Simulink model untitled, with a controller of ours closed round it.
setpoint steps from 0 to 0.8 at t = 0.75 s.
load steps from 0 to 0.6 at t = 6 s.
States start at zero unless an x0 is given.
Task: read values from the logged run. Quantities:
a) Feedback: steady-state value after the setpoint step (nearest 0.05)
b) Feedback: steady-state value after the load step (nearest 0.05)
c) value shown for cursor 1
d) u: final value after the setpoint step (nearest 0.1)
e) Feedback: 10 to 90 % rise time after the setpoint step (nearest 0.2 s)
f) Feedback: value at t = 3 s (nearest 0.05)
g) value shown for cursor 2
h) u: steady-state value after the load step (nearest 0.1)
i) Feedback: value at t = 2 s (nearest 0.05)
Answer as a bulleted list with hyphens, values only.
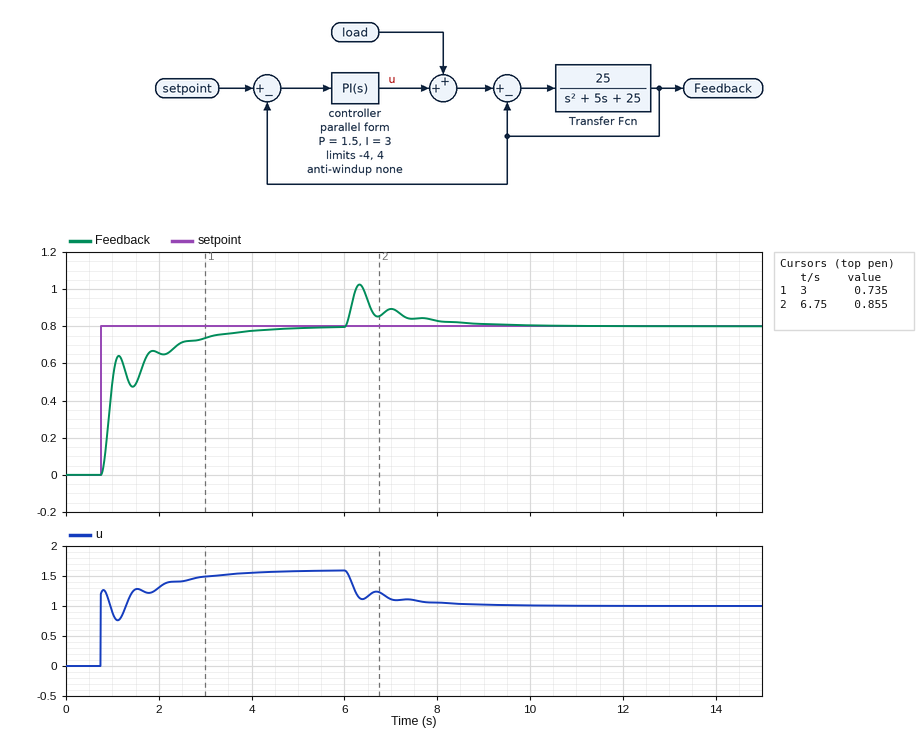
- 0.80
- 0.80
- 0.735
- 1.6
- 1.8 s
- 0.75
- 0.855
- 1.0
- 0.65
